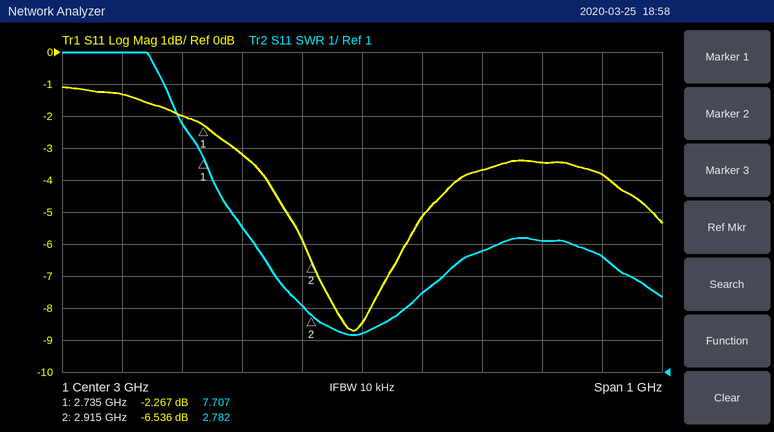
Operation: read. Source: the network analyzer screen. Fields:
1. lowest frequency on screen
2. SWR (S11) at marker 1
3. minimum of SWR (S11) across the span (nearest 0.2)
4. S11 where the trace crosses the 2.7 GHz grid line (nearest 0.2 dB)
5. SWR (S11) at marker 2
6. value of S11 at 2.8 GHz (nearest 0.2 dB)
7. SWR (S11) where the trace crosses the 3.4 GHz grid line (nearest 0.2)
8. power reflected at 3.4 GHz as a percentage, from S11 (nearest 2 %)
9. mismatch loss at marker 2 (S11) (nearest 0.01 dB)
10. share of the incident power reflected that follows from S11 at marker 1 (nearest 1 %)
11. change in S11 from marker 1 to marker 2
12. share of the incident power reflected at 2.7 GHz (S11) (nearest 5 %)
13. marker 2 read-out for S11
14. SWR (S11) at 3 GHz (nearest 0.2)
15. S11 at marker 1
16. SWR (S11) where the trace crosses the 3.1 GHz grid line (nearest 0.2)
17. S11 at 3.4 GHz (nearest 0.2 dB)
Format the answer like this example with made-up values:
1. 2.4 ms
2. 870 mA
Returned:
1. 2.5 GHz
2. 7.707
3. 2.2
4. -2.0 dB
5. 2.782
6. -3.2 dB
7. 4.6
8. 42 %
9. 1.09 dB
10. 59 %
11. -4.269 dB
12. 65 %
13. -6.536 dB
14. 2.2
15. -2.267 dB
16. 3.4
17. -3.8 dB
